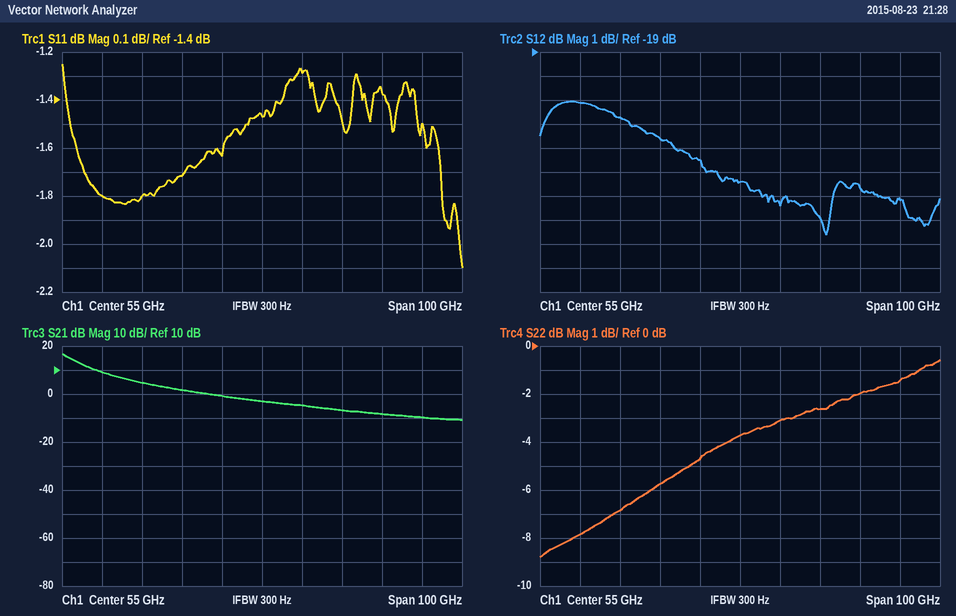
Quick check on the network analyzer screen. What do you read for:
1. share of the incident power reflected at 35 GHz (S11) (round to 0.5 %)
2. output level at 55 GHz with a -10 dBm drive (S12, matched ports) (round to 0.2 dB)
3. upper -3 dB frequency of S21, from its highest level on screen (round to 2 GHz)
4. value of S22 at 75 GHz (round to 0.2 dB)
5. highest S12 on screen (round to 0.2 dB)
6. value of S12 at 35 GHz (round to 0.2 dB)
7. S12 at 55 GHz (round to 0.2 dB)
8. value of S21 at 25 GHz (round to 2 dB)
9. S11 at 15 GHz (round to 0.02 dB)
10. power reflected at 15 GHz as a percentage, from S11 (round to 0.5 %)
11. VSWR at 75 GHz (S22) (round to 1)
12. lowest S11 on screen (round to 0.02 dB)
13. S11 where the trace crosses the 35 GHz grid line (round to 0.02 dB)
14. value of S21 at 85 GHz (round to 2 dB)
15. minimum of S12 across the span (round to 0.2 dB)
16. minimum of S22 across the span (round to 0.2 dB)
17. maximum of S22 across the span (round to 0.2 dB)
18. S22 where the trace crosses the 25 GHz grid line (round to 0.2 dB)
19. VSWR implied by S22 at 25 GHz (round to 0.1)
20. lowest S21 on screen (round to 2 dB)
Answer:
67.5 %
-34.4 dBm
8 GHz
-2.6 dB
-21.0 dB
-22.6 dB
-24.4 dB
4 dB
-1.80 dB
66.0 %
7
-2.10 dB
-1.72 dB
-8 dB
-26.6 dB
-8.8 dB
-0.6 dB
-6.8 dB
2.7
-10 dB
